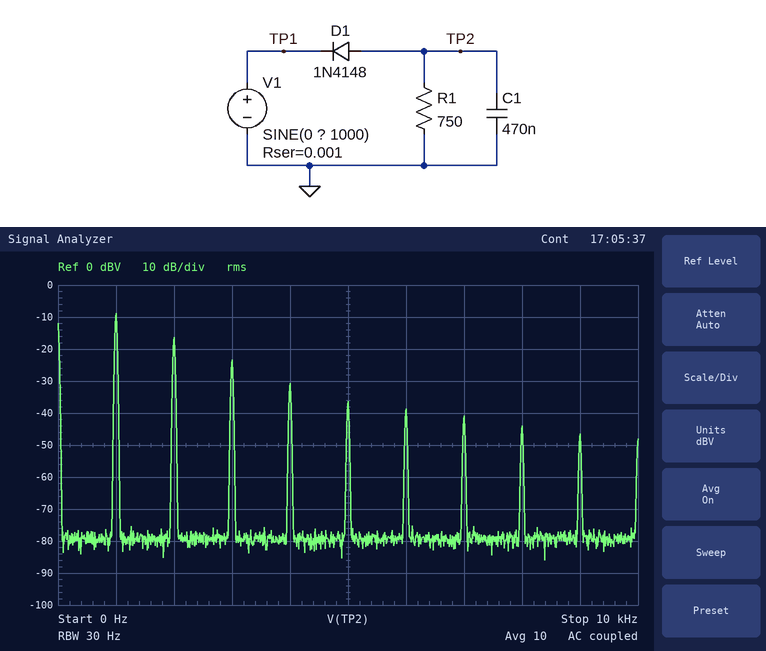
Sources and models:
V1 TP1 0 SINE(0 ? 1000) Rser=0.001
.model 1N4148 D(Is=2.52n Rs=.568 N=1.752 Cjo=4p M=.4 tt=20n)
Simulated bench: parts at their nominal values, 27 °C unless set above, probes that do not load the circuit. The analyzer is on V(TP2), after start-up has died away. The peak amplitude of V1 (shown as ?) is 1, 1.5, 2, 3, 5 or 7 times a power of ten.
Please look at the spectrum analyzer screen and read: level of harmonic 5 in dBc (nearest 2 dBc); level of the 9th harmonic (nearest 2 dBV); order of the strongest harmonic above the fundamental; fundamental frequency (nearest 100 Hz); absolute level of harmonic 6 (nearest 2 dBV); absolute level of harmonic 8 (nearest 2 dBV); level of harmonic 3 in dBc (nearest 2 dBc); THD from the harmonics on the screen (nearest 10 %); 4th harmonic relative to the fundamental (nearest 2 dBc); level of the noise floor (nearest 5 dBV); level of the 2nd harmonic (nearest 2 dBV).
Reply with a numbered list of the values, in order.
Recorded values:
1. -28 dBc
2. -46 dBV
3. 2
4. 1.0 kHz
5. -38 dBV
6. -44 dBV
7. -14 dBc
8. 50 %
9. -22 dBc
10. -80 dBV
11. -16 dBV
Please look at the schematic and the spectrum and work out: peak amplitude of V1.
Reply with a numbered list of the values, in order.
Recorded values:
1. 2 V
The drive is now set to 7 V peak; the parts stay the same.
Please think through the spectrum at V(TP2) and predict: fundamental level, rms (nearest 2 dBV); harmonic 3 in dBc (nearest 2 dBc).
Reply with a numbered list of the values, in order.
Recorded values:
1. 4 dBV
2. -16 dBc
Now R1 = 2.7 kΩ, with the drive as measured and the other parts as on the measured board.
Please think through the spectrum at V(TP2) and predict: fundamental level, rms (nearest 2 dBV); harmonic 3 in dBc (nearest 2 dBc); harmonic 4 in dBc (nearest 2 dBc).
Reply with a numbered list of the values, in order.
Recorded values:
1. -14 dBV
2. -12 dBc
3. -16 dBc
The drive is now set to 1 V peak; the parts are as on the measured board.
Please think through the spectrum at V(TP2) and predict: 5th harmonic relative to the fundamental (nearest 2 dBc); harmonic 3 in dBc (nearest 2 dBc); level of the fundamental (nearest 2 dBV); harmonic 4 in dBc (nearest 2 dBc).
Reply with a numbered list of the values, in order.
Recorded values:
1. -24 dBc
2. -12 dBc
3. -20 dBV
4. -18 dBc
